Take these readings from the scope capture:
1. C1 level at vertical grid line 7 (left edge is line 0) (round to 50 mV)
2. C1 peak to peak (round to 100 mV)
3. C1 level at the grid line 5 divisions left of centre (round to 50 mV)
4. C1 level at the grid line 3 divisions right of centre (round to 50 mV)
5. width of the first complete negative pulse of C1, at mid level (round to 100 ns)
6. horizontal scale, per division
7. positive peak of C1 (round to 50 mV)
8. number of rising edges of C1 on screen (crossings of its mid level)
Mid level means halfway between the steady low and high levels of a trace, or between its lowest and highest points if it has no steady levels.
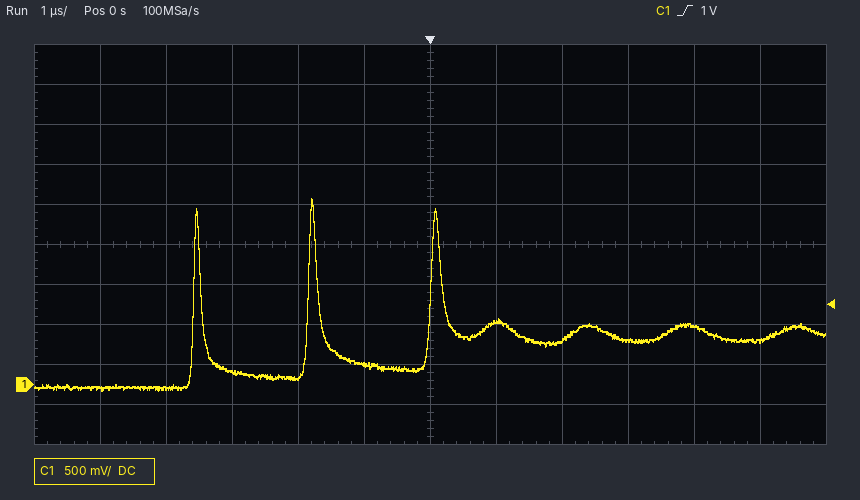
800 mV
2.40 V
-50 mV
550 mV
1.6 µs
1 µs
2.30 V
3
